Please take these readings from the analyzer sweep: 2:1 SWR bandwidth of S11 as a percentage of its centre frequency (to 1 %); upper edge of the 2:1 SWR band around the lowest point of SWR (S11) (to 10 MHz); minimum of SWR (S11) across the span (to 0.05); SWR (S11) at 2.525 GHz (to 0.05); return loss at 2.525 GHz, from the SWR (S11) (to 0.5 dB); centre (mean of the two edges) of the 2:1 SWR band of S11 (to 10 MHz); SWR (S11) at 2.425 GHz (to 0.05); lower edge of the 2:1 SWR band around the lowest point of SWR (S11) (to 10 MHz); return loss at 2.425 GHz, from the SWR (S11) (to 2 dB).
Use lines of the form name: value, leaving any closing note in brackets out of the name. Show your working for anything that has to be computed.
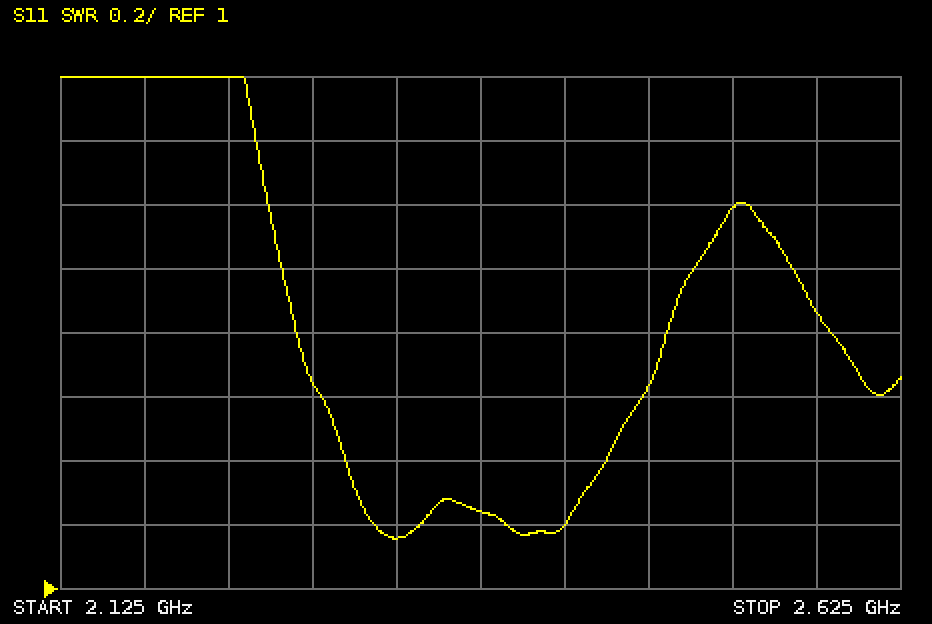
2:1 SWR bandwidth of S11 as a percentage of its centre frequency: 240 MHz / 2.38 GHz ≈ 10 %
upper edge of the 2:1 SWR band around the lowest point of SWR (S11): 2.50 GHz
minimum of SWR (S11) across the span: 1.15
SWR (S11) at 2.525 GHz: 2.20
return loss at 2.525 GHz, from the SWR (S11): −20 log10((2.2 − 1)/(2.2 + 1)) ≈ 8.5 dB
centre (mean of the two edges) of the 2:1 SWR band of S11: 2.38 GHz
SWR (S11) at 2.425 GHz: 1.20
lower edge of the 2:1 SWR band around the lowest point of SWR (S11): 2.26 GHz
return loss at 2.425 GHz, from the SWR (S11): −20 log10((1.2 − 1)/(1.2 + 1)) ≈ 20.8 dB, so 20 dB to the nearest 2 dB
